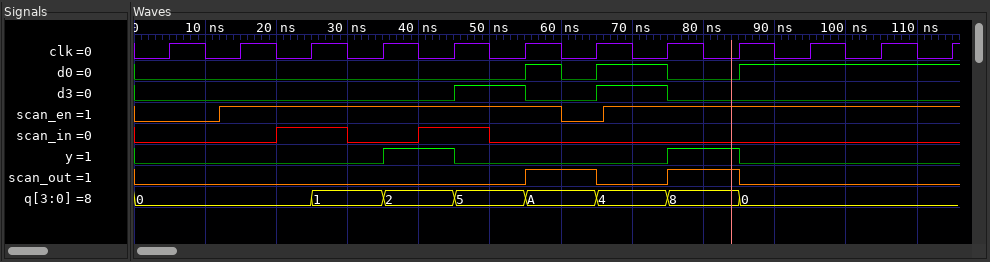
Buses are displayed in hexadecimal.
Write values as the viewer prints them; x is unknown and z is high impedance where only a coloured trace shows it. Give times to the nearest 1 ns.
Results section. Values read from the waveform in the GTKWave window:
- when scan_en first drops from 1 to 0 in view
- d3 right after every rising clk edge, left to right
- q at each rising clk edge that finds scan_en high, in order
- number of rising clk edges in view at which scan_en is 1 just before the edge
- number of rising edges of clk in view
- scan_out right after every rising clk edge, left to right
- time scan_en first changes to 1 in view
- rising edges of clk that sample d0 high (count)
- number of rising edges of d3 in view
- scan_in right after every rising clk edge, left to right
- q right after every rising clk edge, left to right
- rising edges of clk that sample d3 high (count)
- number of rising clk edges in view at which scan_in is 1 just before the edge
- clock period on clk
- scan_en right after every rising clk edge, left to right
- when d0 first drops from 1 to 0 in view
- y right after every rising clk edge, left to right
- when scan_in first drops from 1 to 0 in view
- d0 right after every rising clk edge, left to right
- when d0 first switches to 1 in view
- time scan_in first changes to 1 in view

60 ns
0 0 0 0 1 0 1 0 0 0 0 0
0, 0, 1, 2, 5, 4, 8, 0, 0, 0
10
12
0 0 0 0 0 1 0 1 0 0 0 0
12 ns
4
2
0 0 1 0 1 0 0 0 0 0 0 0
0, 0, 1, 2, 5, A, 4, 8, 0, 0, 0, 0
2
2
10 ns
0 1 1 1 1 1 0 1 1 1 1 1
60 ns
0 0 0 1 0 0 0 1 0 0 0 0
30 ns
0 0 0 0 0 1 1 0 1 1 1 1
55 ns
20 ns
